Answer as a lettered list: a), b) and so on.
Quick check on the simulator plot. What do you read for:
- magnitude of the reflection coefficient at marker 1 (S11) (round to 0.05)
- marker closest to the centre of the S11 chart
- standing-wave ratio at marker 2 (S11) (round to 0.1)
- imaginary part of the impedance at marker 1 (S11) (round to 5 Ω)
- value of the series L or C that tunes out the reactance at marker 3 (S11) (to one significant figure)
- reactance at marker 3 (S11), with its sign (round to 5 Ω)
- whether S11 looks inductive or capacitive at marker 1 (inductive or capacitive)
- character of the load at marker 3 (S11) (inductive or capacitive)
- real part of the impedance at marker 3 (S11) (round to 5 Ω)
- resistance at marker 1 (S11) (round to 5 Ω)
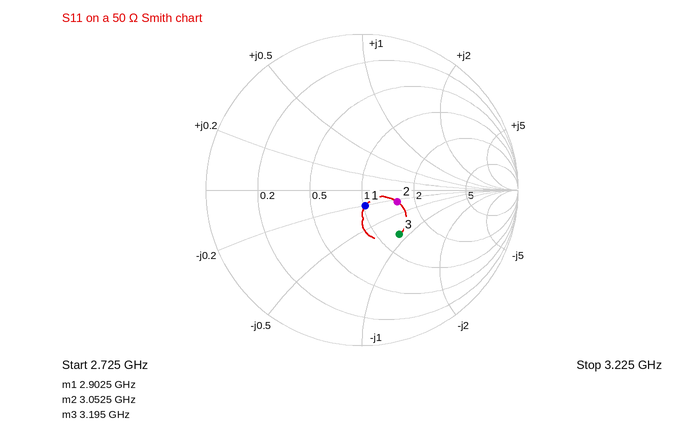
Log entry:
a) 0.10
b) marker 1
c) 1.6
d) -10 Ω
e) 2 nH
f) -45 Ω
g) capacitive
h) capacitive
i) 65 Ω
j) 50 Ω
